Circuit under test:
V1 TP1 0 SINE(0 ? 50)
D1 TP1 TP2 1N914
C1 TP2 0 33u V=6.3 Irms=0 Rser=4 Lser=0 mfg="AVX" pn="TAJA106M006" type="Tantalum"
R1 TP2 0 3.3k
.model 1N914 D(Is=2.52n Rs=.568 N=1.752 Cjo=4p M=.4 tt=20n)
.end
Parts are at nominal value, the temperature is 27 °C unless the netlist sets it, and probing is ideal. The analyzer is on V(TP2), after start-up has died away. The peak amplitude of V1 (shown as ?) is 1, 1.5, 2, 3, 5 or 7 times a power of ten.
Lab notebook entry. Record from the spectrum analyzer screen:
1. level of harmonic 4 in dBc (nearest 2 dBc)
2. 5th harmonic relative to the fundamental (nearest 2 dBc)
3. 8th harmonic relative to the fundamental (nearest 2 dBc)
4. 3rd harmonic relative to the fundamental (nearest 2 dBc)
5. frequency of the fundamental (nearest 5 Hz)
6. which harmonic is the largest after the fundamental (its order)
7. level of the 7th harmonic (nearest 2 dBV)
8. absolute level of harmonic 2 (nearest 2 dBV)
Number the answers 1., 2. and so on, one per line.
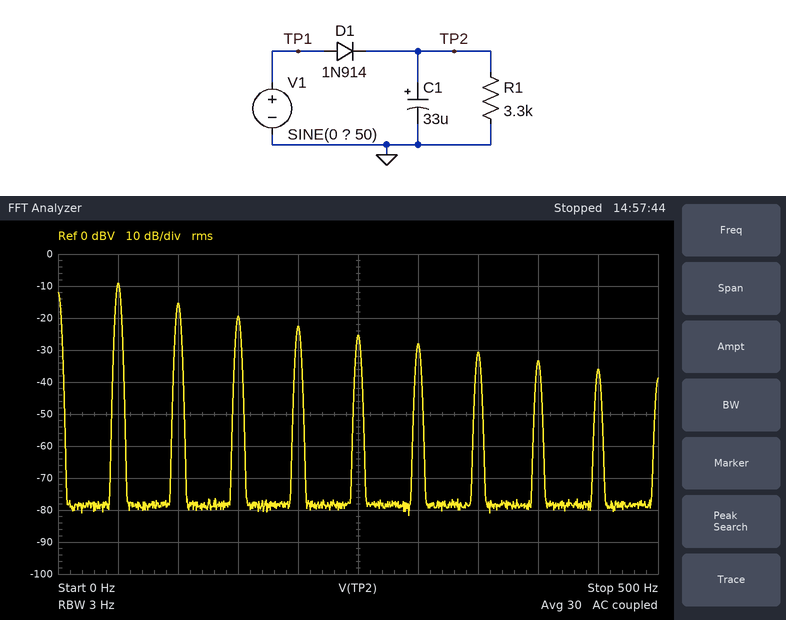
1. -14 dBc
2. -16 dBc
3. -24 dBc
4. -10 dBc
5. 50 Hz
6. 2
7. -30 dBV
8. -16 dBV
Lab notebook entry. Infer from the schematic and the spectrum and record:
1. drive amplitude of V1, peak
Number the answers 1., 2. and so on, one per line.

1. 10 V
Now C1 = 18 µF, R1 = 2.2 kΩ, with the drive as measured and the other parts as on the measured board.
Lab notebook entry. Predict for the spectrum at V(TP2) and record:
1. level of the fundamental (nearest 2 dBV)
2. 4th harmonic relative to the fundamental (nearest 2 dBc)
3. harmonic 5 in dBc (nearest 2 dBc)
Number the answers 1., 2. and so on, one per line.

1. -2 dBV
2. -16 dBc
3. -20 dBc
